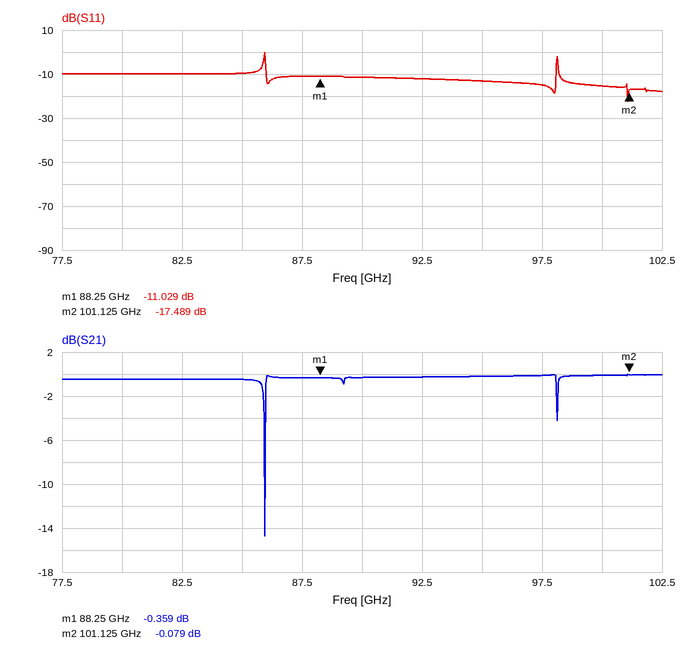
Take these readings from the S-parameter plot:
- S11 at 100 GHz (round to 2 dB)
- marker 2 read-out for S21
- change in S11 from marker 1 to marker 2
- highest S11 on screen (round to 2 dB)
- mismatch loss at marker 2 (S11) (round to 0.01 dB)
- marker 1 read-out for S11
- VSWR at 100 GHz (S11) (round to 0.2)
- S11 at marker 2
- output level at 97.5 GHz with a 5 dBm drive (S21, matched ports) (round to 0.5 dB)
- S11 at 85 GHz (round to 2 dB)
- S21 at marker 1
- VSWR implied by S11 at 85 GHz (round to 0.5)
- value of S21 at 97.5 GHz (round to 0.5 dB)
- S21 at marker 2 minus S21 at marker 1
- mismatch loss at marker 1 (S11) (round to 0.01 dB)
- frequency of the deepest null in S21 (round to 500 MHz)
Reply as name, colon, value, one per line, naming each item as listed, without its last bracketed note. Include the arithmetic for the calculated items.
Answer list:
S11 at 100 GHz: -16 dB
marker 2 read-out for S21: -0.079 dB
change in S11 from marker 1 to marker 2: -17.489 − (-11.029) = -6.460 dB
highest S11 on screen: 0 dB
mismatch loss at marker 2 (S11): −10 log10(1 − 10^(-17.489/10)) ≈ 0.08 dB
marker 1 read-out for S11: -11.029 dB
VSWR at 100 GHz (S11): |Γ| = 10^(-16/20) = 0.1585; VSWR = (1 + 0.1585)/(1 − 0.1585) ≈ 1.4
S11 at marker 2: -17.489 dB
output level at 97.5 GHz with a 5 dBm drive (S21, matched ports): 5 dBm + (0.0 dB) = 5.0 dBm
S11 at 85 GHz: -10 dB
S21 at marker 1: -0.359 dB
VSWR implied by S11 at 85 GHz: |Γ| = 10^(-10/20) = 0.3162; VSWR = (1 + 0.3162)/(1 − 0.3162) ≈ 1.92, so 2.0 to the nearest 0.5
value of S21 at 97.5 GHz: 0.0 dB
S21 at marker 2 minus S21 at marker 1: -0.079 − (-0.359) = 0.280 dB
mismatch loss at marker 1 (S11): −10 log10(1 − 10^(-11.029/10)) ≈ 0.36 dB
frequency of the deepest null in S21: 86.0 GHz
